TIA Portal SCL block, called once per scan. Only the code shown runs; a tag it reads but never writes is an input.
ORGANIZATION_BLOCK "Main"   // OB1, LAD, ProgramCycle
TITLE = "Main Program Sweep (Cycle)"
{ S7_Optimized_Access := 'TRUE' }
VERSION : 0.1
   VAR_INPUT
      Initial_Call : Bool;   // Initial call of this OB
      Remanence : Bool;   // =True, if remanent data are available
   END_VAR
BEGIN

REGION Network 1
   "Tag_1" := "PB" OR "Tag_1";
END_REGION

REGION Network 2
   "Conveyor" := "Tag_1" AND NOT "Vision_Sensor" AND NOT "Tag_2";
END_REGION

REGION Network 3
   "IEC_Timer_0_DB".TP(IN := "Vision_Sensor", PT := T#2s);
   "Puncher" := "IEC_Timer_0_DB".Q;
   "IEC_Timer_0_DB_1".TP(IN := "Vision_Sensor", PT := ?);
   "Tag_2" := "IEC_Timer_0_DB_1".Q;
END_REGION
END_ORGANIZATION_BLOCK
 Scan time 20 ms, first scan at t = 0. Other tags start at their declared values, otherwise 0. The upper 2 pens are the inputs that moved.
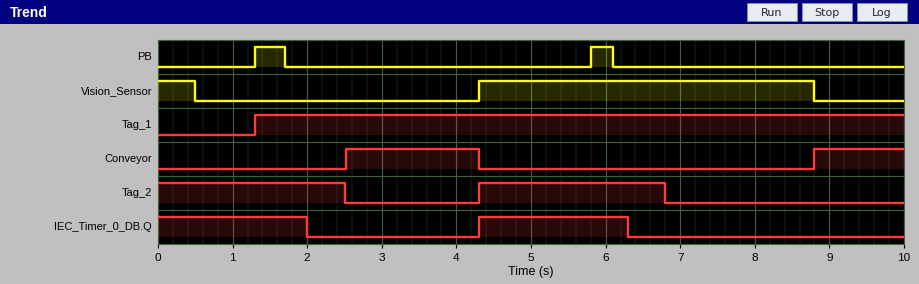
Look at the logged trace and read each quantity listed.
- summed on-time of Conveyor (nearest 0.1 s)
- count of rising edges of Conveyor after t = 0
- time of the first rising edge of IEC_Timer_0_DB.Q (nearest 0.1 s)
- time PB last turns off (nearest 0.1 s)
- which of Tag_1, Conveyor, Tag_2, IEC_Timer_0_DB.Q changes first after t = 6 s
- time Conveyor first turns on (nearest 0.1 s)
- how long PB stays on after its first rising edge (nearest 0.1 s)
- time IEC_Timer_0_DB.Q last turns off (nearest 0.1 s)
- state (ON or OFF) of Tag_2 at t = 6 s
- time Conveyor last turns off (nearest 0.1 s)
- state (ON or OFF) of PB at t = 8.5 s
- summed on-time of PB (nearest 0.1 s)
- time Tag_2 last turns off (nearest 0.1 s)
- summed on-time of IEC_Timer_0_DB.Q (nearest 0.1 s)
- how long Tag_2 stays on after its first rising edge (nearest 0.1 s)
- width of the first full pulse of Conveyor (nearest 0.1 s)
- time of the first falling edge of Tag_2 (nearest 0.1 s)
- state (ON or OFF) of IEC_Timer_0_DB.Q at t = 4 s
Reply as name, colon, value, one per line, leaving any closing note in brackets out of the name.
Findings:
summed on-time of Conveyor: 3.0 s
count of rising edges of Conveyor after t = 0: 2
time of the first rising edge of IEC_Timer_0_DB.Q: 4.3 s
time PB last turns off: 6.1 s
which of Tag_1, Conveyor, Tag_2, IEC_Timer_0_DB.Q changes first after t = 6 s: IEC_Timer_0_DB.Q
time Conveyor first turns on: 2.5 s
how long PB stays on after its first rising edge: 0.4 s
time IEC_Timer_0_DB.Q last turns off: 6.3 s
state (ON or OFF) of Tag_2 at t = 6 s: ON
time Conveyor last turns off: 4.3 s
state (ON or OFF) of PB at t = 8.5 s: OFF
summed on-time of PB: 0.7 s
time Tag_2 last turns off: 6.8 s
summed on-time of IEC_Timer_0_DB.Q: 4.0 s
how long Tag_2 stays on after its first rising edge: 2.5 s
width of the first full pulse of Conveyor: 1.8 s
time of the first falling edge of Tag_2: 2.5 s
state (ON or OFF) of IEC_Timer_0_DB.Q at t = 4 s: OFF
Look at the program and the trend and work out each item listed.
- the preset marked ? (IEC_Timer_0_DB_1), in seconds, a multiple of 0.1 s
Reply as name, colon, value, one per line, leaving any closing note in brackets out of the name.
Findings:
the preset marked ? (IEC_Timer_0_DB_1), in seconds, a multiple of 0.1 s: 2.5 s
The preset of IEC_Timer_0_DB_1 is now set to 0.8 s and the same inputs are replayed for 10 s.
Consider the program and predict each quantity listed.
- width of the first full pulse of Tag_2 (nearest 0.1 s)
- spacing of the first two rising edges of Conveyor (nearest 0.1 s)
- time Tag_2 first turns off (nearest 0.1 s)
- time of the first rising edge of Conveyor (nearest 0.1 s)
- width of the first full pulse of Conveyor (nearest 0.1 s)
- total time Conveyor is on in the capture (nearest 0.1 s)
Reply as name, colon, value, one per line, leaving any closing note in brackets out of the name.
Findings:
width of the first full pulse of Tag_2: 0.8 s
spacing of the first two rising edges of Conveyor: 7.5 s
time Tag_2 first turns off: 0.8 s
time of the first rising edge of Conveyor: 1.3 s
width of the first full pulse of Conveyor: 3.0 s
total time Conveyor is on in the capture: 4.2 s
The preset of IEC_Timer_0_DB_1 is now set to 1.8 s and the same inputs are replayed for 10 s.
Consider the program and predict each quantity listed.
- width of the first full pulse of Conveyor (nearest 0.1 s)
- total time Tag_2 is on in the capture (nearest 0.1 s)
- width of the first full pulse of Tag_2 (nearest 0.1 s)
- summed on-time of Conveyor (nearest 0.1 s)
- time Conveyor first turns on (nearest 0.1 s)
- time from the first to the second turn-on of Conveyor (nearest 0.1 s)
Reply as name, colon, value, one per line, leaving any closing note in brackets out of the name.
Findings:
width of the first full pulse of Conveyor: 2.5 s
total time Tag_2 is on in the capture: 3.6 s
width of the first full pulse of Tag_2: 1.8 s
summed on-time of Conveyor: 3.7 s
time Conveyor first turns on: 1.8 s
time from the first to the second turn-on of Conveyor: 7.0 s
